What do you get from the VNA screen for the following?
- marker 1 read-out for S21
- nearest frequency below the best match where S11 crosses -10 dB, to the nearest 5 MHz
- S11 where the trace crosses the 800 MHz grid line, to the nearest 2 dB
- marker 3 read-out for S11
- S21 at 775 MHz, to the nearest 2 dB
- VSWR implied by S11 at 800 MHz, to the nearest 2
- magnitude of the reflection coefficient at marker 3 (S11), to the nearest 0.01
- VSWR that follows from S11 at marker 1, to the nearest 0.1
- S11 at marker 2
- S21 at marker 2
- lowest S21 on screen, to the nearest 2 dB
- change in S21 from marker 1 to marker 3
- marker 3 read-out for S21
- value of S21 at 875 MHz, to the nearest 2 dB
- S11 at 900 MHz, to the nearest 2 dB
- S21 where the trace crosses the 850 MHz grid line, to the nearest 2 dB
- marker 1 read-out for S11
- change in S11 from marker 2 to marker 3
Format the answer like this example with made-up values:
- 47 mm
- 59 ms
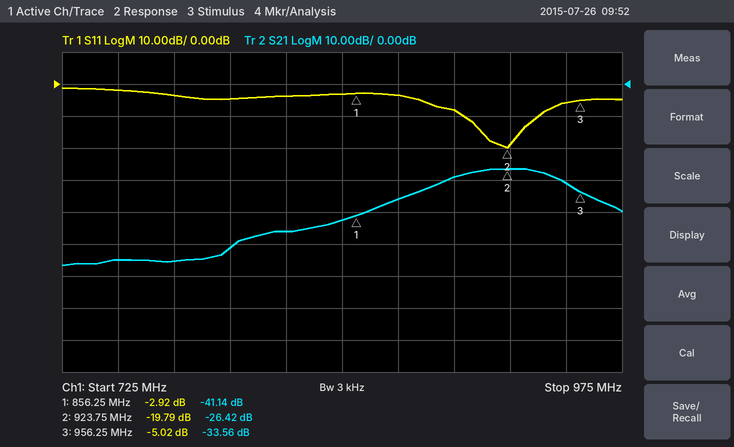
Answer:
- -41.14 dB
- 905 MHz
- -4 dB
- -5.02 dB
- -56 dB
- 4
- 0.56
- 6.0
- -19.79 dB
- -26.42 dB
- -56 dB
- 7.58 dB
- -33.56 dB
- -36 dB
- -8 dB
- -42 dB
- -2.92 dB
- 14.77 dB
